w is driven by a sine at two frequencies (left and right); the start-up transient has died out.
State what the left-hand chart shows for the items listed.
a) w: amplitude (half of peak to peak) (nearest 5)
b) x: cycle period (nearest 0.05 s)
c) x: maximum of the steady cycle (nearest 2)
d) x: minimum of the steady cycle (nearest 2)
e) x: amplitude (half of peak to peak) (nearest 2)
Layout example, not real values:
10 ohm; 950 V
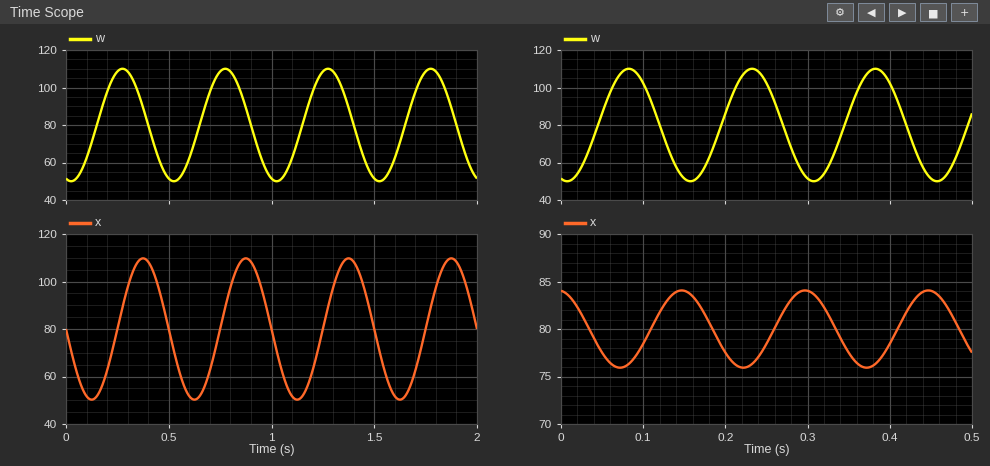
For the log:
30; 0.50 s; 110; 50; 30
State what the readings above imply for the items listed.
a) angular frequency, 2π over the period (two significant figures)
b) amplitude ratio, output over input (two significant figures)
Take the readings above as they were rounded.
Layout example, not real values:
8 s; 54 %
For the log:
13 rad/s; 1.0
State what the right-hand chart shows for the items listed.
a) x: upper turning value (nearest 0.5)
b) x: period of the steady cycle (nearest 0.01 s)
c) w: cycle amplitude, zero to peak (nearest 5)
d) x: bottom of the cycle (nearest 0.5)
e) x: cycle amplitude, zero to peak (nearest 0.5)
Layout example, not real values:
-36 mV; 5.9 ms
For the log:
84.0; 0.15 s; 30; 76.0; 4.0
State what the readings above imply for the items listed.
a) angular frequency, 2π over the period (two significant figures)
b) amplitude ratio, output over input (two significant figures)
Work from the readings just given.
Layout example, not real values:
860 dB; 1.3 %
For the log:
42 rad/s; 0.13
